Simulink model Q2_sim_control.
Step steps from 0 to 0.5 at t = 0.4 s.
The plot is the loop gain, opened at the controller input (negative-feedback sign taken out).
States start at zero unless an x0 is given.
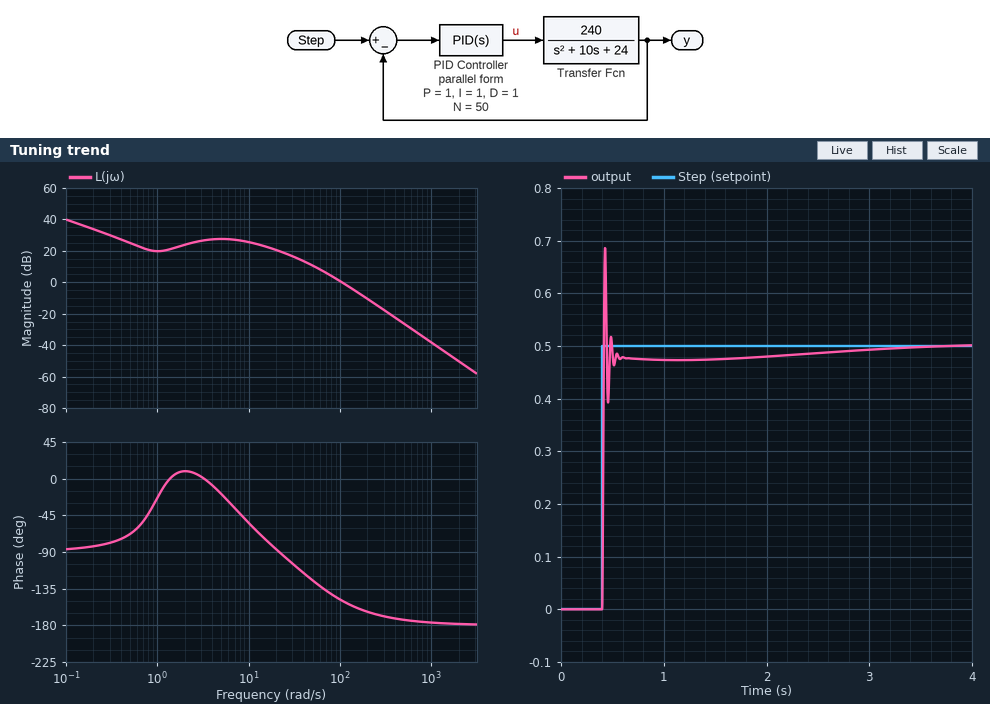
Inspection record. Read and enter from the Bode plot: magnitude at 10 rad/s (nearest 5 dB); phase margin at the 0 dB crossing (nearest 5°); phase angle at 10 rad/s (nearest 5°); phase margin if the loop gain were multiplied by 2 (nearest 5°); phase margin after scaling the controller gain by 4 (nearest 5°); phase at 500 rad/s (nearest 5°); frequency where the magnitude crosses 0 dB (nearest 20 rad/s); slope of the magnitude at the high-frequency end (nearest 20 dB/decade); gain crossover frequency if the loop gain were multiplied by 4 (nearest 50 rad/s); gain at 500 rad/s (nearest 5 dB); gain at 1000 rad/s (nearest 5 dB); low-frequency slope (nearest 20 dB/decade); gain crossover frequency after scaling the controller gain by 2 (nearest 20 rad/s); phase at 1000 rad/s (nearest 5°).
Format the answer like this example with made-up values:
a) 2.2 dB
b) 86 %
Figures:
a) 25 dB
b) 30°
c) -55°
d) 20°
e) 15°
f) -175°
g) 100 rad/s
h) -40 dB/decade
i) 200 rad/s
j) -25 dB
k) -40 dB
l) -20 dB/decade
m) 160 rad/s
n) -175°
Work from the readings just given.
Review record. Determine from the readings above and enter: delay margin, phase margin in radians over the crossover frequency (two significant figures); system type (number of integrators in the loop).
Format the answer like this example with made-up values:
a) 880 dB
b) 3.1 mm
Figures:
a) 0.0052 s
b) 1
